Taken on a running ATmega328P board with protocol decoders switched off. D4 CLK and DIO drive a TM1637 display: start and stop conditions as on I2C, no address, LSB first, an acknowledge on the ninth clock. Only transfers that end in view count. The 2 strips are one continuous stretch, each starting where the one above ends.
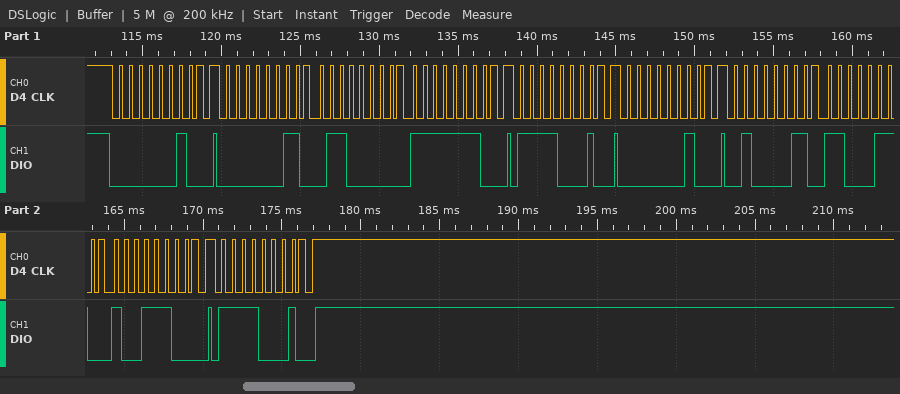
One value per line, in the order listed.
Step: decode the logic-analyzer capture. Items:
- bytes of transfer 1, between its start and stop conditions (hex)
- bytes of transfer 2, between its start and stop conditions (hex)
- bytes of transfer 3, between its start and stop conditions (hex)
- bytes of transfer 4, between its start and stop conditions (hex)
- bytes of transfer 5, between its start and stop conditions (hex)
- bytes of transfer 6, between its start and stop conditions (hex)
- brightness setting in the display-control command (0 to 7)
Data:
40
C0 06 7F
8F
40
C2 63 39
8F
7
